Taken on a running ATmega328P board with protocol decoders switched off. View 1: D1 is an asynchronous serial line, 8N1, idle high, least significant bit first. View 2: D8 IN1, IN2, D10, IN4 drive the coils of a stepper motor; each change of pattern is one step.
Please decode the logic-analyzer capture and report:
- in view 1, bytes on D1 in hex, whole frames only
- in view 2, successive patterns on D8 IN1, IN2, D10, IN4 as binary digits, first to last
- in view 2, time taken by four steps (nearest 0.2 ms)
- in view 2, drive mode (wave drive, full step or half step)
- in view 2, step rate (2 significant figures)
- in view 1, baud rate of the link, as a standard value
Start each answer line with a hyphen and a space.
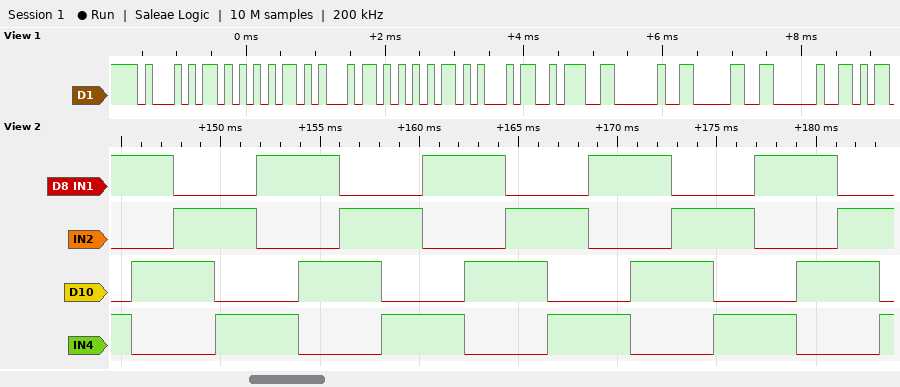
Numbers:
- 0x51 0x55 0x45 0x55 0x45 0x3A 0x20 0x30 0x20
- 1001 1010 0110 0101 1001 1010 0110 0101 1001 1010 0110 0101 1001 1010 0110 0101 1001 1010 0110 0101
- 8.4 ms
- full step
- 480 steps/s
- 9600 baud
